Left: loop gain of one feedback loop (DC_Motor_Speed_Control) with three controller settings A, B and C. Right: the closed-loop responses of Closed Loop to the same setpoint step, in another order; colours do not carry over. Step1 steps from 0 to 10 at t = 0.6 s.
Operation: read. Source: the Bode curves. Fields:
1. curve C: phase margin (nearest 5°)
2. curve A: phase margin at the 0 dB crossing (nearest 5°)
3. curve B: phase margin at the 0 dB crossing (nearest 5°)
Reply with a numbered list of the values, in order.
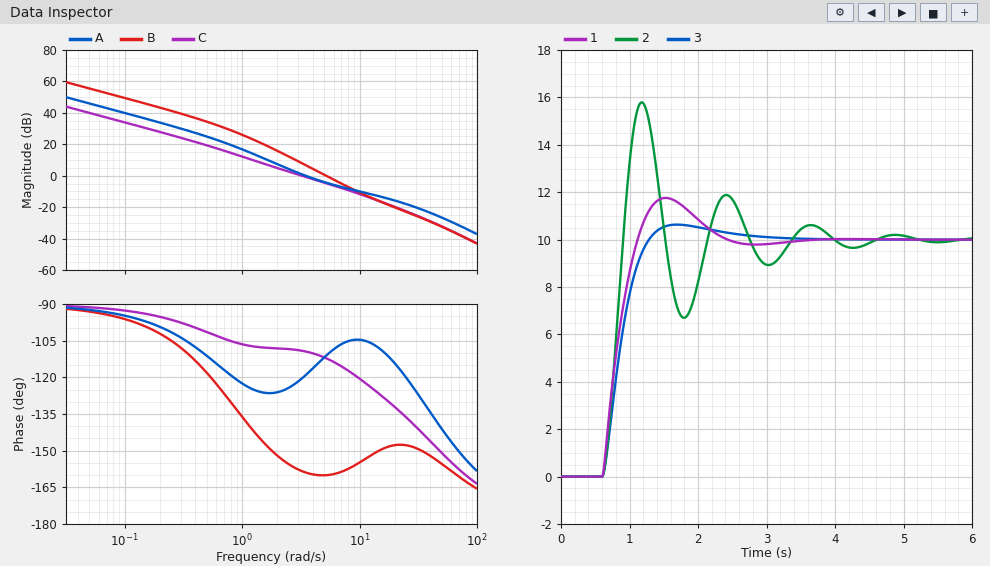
1. 70°
2. 60°
3. 20°
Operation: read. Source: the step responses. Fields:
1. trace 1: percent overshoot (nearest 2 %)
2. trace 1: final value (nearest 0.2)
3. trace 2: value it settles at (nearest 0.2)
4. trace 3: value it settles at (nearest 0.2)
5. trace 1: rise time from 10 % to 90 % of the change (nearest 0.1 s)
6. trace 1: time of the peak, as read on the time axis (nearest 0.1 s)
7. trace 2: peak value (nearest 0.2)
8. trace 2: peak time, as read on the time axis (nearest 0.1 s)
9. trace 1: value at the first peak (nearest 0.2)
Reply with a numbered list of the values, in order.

1. 18 %
2. 10.0
3. 10.0
4. 10.0
5. 0.4 s
6. 1.5 s
7. 15.8
8. 1.2 s
9. 11.8
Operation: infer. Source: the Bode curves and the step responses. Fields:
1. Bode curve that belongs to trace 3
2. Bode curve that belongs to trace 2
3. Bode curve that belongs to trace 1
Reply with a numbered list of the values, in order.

1. C
2. B
3. A
